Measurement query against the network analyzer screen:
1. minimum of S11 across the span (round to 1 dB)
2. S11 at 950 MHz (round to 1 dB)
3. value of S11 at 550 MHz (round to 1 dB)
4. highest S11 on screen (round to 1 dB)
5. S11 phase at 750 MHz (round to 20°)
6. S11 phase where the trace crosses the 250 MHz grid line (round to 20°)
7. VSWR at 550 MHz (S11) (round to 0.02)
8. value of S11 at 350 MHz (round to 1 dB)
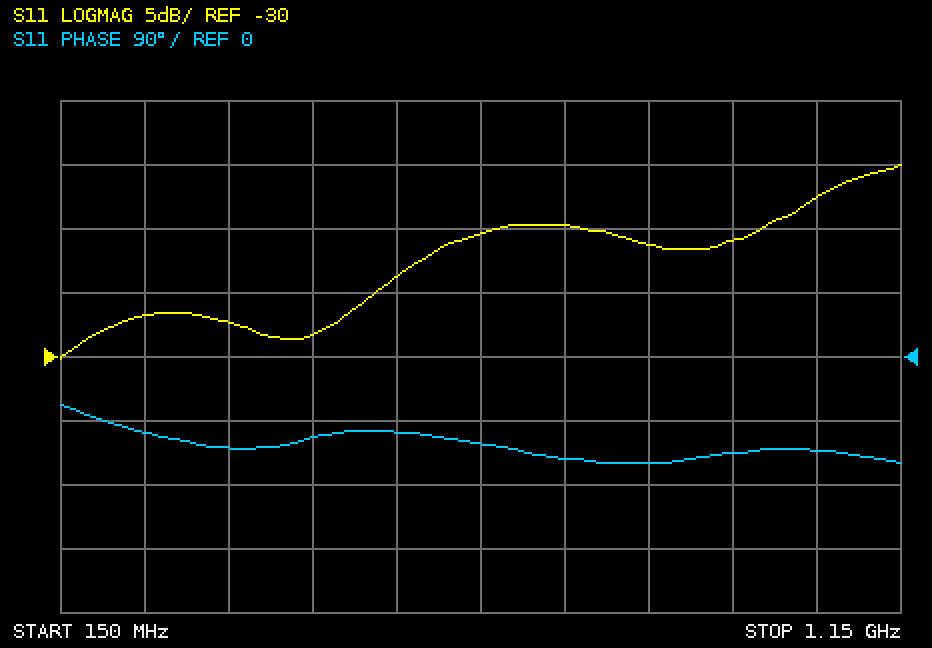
-30 dB
-21 dB
-24 dB
-15 dB
-140°
-100°
1.14
-27 dB
